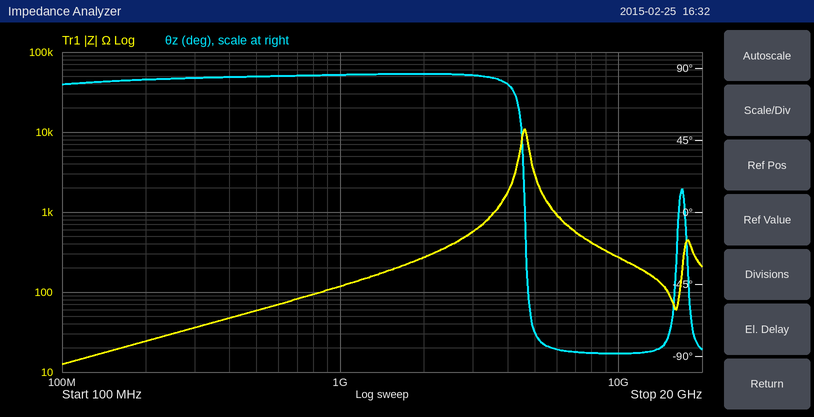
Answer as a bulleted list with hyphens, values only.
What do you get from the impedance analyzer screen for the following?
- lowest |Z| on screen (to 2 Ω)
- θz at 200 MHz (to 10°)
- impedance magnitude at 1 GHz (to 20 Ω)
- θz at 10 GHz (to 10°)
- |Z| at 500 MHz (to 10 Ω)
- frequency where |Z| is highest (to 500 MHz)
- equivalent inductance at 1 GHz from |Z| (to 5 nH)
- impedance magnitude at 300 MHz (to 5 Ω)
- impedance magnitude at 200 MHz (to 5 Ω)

- 12 Ω
- 80°
- 120 Ω
- -90°
- 60 Ω
- 4.5 GHz
- 20 nH
- 35 Ω
- 25 Ω
